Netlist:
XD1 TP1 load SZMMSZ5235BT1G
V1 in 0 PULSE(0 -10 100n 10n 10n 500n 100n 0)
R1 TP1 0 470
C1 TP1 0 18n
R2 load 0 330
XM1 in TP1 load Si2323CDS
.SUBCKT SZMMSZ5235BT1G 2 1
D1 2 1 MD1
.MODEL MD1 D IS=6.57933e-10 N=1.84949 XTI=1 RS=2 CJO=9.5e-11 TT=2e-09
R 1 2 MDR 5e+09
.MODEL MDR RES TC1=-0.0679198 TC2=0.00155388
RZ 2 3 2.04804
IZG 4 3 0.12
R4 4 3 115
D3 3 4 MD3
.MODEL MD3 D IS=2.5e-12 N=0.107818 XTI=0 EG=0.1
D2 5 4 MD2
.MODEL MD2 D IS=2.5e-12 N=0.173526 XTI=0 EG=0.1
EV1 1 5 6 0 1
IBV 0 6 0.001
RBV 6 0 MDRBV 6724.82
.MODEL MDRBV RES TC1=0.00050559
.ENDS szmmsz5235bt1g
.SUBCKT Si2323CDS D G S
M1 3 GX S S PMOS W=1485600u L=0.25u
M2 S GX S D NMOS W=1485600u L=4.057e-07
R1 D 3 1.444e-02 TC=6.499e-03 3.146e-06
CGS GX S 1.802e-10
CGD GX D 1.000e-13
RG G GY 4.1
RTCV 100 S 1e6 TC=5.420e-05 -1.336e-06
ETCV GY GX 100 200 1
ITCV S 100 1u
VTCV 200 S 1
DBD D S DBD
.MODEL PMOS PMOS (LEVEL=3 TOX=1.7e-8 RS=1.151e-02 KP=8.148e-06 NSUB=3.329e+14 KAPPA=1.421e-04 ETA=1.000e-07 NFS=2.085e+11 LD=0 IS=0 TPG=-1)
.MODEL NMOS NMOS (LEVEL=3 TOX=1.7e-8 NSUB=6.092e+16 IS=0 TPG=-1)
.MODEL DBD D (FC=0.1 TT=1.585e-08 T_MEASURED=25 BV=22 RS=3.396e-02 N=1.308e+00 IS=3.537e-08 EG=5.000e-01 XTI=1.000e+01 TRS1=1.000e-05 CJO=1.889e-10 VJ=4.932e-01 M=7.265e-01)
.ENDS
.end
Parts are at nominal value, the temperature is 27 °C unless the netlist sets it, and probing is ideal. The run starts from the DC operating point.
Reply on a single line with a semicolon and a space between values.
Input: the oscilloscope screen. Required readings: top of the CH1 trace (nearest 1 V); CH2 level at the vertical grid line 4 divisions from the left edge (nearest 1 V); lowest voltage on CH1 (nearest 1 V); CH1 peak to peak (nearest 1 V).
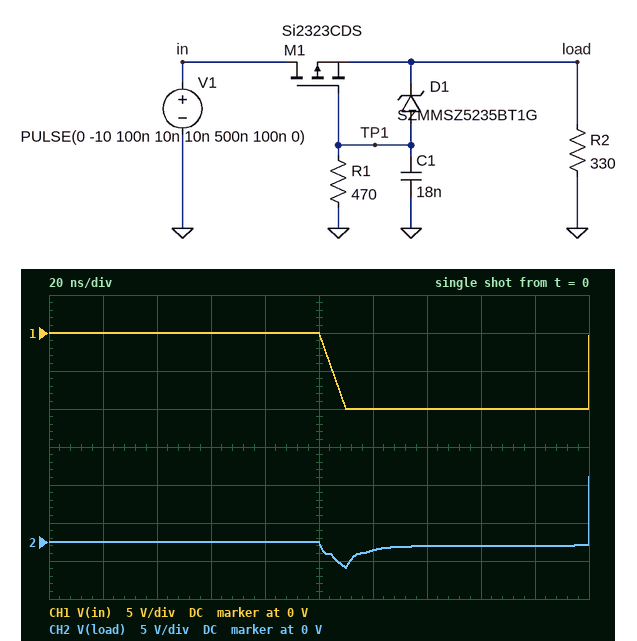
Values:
0 V; 0 V; -10 V; 10 V
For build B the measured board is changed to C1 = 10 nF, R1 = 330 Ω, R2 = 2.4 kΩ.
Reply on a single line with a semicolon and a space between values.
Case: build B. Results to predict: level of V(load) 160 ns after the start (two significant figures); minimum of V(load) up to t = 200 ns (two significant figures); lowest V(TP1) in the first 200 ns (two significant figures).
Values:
-1.2 V; -3.6 V; -1.5 V
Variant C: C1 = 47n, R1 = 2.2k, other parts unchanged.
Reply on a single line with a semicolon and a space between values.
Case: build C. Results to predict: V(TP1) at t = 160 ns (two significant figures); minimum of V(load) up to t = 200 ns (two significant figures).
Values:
-370 mV; -3.2 V
